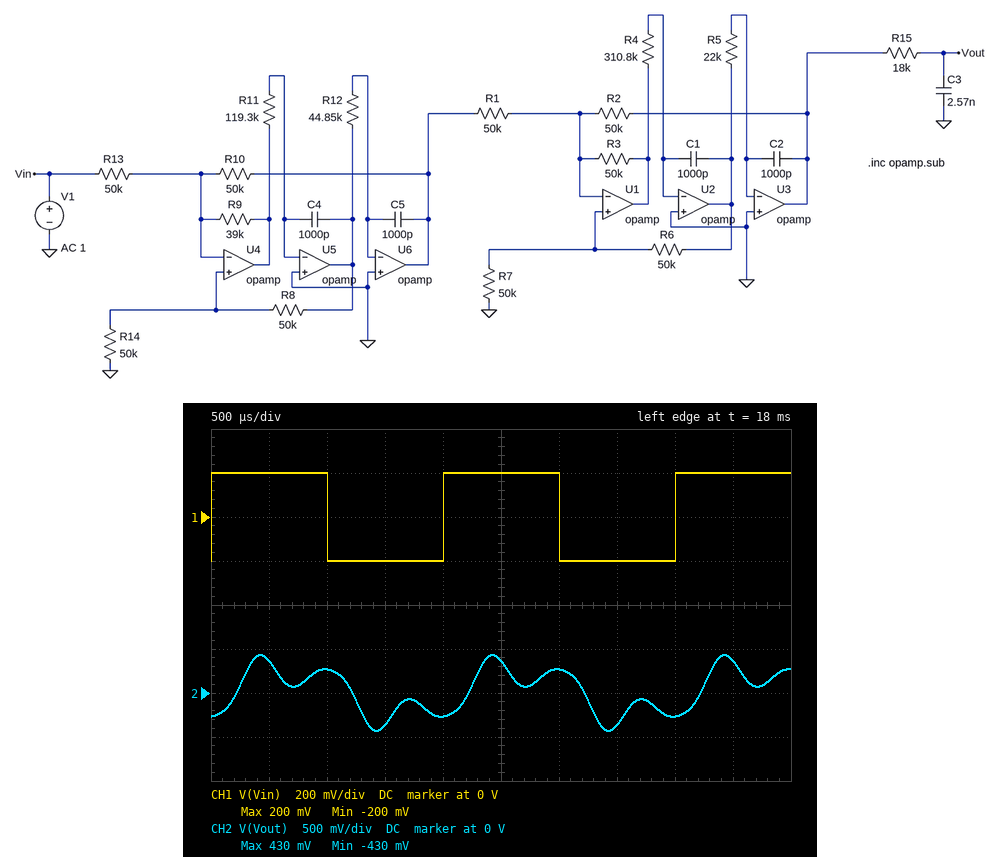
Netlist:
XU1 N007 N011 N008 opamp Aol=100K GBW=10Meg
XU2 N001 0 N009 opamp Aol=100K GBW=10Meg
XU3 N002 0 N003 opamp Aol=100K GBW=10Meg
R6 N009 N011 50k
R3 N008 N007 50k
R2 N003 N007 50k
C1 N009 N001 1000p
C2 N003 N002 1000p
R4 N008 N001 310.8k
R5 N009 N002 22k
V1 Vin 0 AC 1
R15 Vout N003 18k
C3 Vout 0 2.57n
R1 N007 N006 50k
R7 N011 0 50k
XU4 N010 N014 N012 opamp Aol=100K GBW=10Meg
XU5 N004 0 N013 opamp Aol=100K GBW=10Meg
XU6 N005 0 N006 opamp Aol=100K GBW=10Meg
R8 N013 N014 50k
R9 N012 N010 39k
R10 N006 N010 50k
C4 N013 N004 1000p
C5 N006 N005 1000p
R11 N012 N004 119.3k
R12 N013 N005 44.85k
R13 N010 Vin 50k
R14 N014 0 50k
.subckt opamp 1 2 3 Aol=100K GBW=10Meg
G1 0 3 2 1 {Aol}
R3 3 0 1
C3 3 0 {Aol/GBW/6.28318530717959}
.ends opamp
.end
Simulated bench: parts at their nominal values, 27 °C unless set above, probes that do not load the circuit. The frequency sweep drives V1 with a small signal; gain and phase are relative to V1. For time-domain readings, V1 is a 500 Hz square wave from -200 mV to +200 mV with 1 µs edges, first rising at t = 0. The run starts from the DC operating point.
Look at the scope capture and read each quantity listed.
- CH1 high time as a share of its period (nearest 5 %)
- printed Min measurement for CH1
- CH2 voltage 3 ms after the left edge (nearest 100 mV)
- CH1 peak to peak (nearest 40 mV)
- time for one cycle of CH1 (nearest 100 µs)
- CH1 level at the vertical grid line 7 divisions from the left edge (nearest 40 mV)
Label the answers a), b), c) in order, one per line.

a) 50 %
b) -200 mV
c) 300 mV
d) 400 mV
e) 2.0 ms
f) -200 mV
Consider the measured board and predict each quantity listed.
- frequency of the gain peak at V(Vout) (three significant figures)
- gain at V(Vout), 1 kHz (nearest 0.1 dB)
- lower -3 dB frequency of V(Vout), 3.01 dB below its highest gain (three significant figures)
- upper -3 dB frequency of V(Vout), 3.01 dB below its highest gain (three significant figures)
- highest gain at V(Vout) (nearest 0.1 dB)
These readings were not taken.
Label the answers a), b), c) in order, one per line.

a) 1.77 kHz
b) 3.3 dB
c) 1.30 kHz
d) 2.08 kHz
e) 8.6 dB
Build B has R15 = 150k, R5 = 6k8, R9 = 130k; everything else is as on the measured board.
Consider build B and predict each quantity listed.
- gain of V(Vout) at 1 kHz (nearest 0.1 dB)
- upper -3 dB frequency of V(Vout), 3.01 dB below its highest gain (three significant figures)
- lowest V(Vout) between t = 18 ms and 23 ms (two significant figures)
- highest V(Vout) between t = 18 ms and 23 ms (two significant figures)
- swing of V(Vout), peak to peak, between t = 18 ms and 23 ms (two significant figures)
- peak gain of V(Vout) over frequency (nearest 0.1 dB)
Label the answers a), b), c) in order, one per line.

a) -7.4 dB
b) 429 Hz
c) -170 mV
d) 170 mV
e) 340 mV
f) 0 dB
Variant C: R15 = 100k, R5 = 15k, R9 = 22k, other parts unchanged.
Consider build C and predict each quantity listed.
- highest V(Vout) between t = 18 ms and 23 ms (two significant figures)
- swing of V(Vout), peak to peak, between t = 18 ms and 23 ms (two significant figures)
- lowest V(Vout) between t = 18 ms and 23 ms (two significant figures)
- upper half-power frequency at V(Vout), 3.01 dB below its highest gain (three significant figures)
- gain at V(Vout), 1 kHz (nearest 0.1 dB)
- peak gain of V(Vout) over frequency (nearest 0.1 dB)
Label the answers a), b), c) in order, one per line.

a) 190 mV
b) 380 mV
c) -190 mV
d) 1.42 kHz
e) -1.9 dB
f) 0 dB
